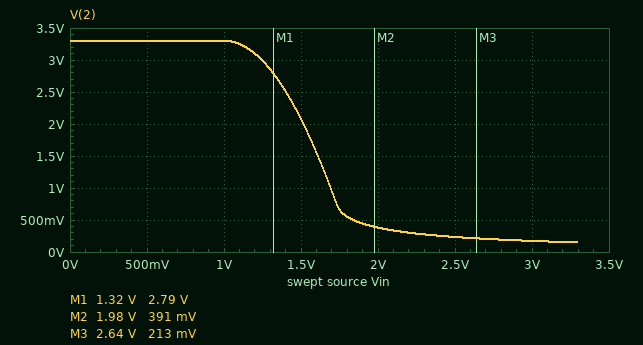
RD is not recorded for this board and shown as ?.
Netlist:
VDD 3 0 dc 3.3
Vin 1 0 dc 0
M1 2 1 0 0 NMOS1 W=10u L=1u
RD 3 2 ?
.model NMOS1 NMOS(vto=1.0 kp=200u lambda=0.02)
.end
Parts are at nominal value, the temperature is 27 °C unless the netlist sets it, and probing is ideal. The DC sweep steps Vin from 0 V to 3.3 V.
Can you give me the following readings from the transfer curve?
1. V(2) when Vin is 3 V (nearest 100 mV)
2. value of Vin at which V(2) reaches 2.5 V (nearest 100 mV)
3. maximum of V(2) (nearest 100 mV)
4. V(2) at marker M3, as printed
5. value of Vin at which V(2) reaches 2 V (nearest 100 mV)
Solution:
200 mV
1.4 V
3.3 V
213 mV
1.5 V
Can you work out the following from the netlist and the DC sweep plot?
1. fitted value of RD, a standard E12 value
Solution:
4.7 kΩ
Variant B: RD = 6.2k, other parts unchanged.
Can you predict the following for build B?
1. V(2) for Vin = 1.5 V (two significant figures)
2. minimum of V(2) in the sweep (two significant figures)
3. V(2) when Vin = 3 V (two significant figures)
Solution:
1.7 V
110 mV
130 mV
